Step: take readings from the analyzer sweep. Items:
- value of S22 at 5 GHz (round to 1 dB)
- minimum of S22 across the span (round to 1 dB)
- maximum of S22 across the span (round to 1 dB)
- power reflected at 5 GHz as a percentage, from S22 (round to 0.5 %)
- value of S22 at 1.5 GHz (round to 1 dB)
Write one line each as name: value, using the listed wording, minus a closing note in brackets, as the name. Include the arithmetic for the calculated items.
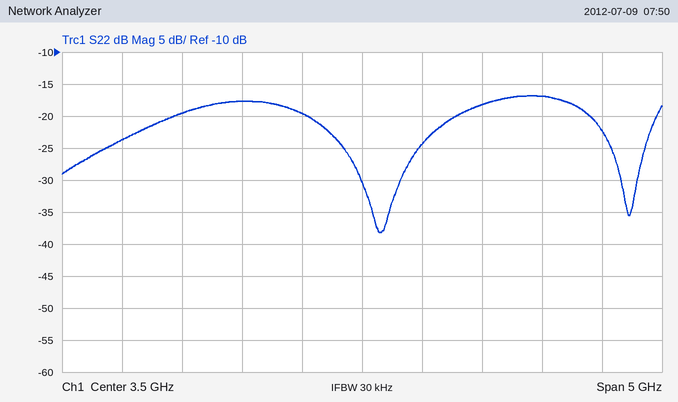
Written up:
value of S22 at 5 GHz: -17 dB
minimum of S22 across the span: -38 dB
maximum of S22 across the span: -17 dB
power reflected at 5 GHz as a percentage, from S22: 10^(-17/10) ≈ 2.0 %
value of S22 at 1.5 GHz: -24 dB
